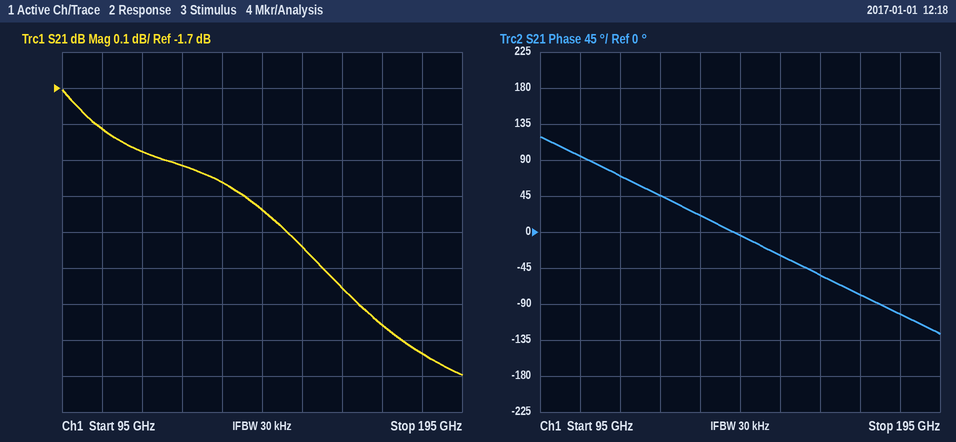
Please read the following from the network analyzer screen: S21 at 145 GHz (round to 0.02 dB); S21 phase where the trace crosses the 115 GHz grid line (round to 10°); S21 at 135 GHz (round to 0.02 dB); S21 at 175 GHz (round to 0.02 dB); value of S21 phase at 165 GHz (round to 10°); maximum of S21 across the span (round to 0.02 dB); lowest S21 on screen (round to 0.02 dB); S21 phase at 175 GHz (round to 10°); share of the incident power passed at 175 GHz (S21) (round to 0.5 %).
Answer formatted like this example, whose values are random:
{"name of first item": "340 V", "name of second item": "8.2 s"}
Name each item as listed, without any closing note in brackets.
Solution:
{"S21 at 145 GHz": "-2.04 dB", "S21 phase where the trace crosses the 115 GHz grid line": "70°", "S21 at 135 GHz": "-1.96 dB", "S21 at 175 GHz": "-2.36 dB", "value of S21 phase at 165 GHz": "-50°", "maximum of S21 across the span": "-1.70 dB", "lowest S21 on screen": "-2.50 dB", "S21 phase at 175 GHz": "-80°", "share of the incident power passed at 175 GHz (S21)": "58.0 %"}
